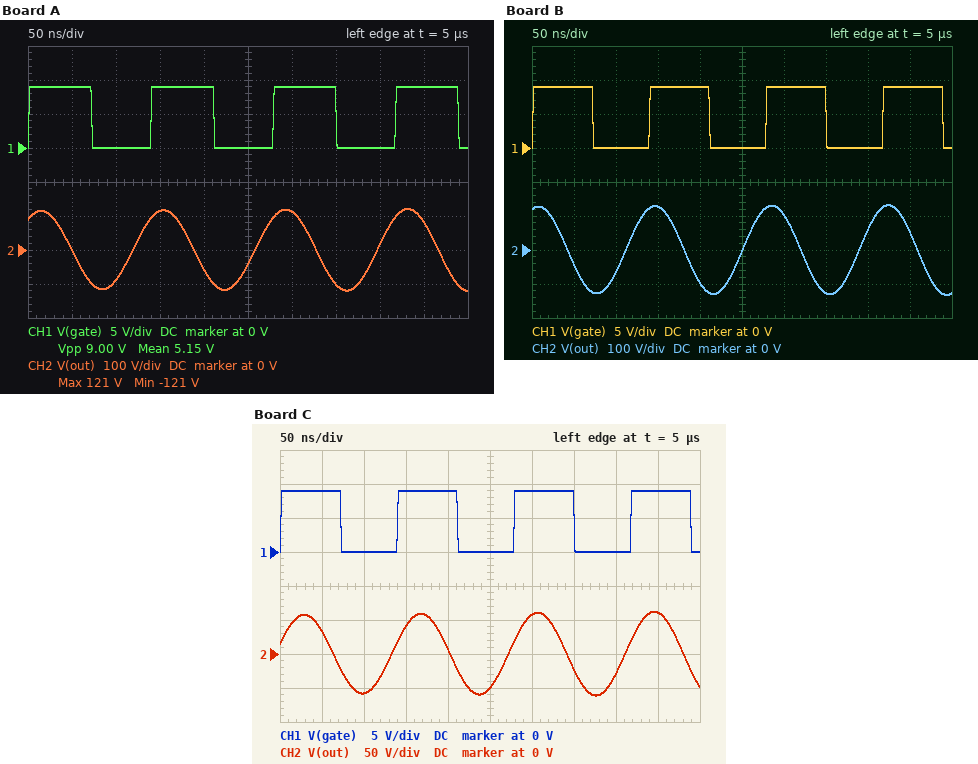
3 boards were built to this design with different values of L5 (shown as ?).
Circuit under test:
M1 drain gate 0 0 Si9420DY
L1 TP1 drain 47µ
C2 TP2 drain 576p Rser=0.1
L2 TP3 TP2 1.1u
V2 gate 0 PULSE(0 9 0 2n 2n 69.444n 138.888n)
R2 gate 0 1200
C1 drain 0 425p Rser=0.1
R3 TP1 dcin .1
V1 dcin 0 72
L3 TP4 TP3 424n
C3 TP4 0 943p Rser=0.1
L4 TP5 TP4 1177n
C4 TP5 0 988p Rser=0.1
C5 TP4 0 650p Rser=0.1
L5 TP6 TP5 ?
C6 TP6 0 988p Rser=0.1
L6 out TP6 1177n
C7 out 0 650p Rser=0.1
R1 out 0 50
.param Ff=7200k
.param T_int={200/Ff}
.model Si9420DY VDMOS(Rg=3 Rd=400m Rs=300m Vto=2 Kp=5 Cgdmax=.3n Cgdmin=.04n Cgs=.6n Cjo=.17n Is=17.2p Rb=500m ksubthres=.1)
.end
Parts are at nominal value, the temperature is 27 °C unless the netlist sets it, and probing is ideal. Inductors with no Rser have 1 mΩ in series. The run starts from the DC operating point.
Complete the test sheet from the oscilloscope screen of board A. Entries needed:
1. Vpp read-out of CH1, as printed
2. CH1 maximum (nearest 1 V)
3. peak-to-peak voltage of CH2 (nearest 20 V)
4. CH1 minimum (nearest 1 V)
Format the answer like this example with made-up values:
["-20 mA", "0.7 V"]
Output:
["9.00 V", "9 V", "240 V", "0 V"]
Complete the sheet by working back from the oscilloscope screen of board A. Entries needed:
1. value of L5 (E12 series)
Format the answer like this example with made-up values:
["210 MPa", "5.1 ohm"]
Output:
["2.2 µH"]
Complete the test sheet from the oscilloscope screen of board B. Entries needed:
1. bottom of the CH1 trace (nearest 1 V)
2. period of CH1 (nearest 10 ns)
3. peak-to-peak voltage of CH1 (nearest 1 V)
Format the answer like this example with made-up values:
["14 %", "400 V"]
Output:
["0 V", "140 ns", "9 V"]
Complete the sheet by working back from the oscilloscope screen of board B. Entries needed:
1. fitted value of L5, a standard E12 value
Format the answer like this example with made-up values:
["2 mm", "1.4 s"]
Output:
["1.8 µH"]
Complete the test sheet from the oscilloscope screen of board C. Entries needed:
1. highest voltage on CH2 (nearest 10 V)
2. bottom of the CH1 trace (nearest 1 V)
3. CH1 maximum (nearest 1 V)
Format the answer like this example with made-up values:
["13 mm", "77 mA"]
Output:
["60 V", "0 V", "9 V"]
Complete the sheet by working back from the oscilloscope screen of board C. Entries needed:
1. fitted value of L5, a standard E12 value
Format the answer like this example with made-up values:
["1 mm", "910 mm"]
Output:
["3.9 µH"]
